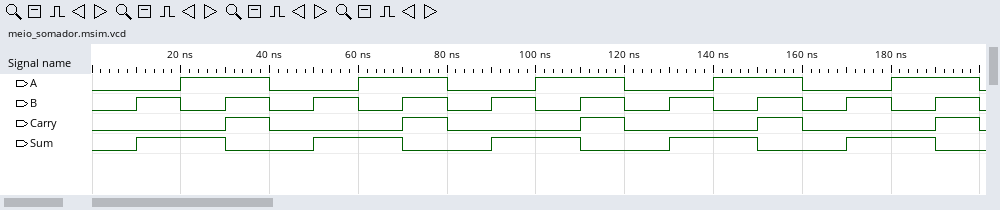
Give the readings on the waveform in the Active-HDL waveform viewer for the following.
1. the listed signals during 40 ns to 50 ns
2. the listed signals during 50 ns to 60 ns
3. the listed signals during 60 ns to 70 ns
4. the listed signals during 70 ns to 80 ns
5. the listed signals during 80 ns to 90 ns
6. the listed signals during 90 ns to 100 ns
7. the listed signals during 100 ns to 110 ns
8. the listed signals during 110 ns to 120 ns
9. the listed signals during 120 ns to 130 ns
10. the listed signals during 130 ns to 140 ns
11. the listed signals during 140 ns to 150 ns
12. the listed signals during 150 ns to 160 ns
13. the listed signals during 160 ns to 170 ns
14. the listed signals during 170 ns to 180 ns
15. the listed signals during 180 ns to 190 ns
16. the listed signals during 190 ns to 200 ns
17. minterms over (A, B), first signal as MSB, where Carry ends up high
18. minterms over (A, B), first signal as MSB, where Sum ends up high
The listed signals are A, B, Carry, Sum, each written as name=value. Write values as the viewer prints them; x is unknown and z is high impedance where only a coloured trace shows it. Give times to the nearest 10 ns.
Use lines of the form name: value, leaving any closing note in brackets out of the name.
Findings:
the listed signals during 40 ns to 50 ns: A=0, B=0, Carry=0, Sum=0
the listed signals during 50 ns to 60 ns: A=0, B=1, Carry=0, Sum=1
the listed signals during 60 ns to 70 ns: A=1, B=0, Carry=0, Sum=1
the listed signals during 70 ns to 80 ns: A=1, B=1, Carry=1, Sum=0
the listed signals during 80 ns to 90 ns: A=0, B=0, Carry=0, Sum=0
the listed signals during 90 ns to 100 ns: A=0, B=1, Carry=0, Sum=1
the listed signals during 100 ns to 110 ns: A=1, B=0, Carry=0, Sum=1
the listed signals during 110 ns to 120 ns: A=1, B=1, Carry=1, Sum=0
the listed signals during 120 ns to 130 ns: A=0, B=0, Carry=0, Sum=0
the listed signals during 130 ns to 140 ns: A=0, B=1, Carry=0, Sum=1
the listed signals during 140 ns to 150 ns: A=1, B=0, Carry=0, Sum=1
the listed signals during 150 ns to 160 ns: A=1, B=1, Carry=1, Sum=0
the listed signals during 160 ns to 170 ns: A=0, B=0, Carry=0, Sum=0
the listed signals during 170 ns to 180 ns: A=0, B=1, Carry=0, Sum=1
the listed signals during 180 ns to 190 ns: A=1, B=0, Carry=0, Sum=1
the listed signals during 190 ns to 200 ns: A=1, B=1, Carry=1, Sum=0
minterms over (A, B), first signal as MSB, where Carry ends up high: 3
minterms over (A, B), first signal as MSB, where Sum ends up high: 1, 2
